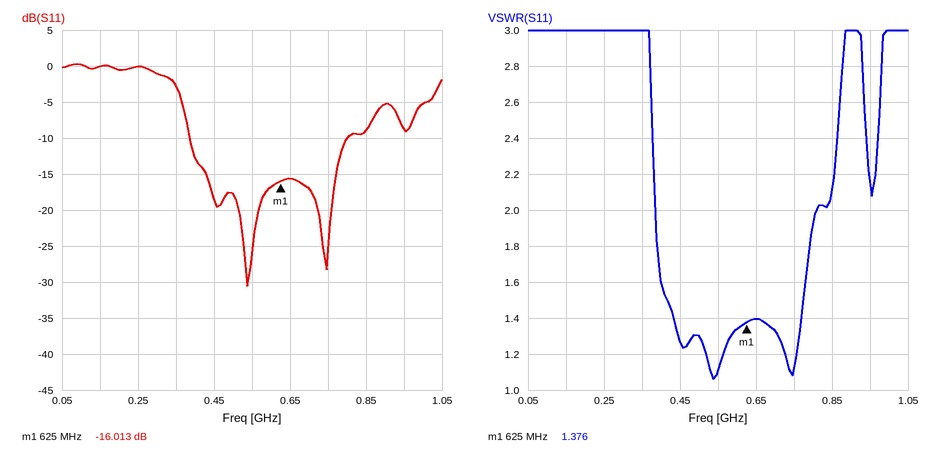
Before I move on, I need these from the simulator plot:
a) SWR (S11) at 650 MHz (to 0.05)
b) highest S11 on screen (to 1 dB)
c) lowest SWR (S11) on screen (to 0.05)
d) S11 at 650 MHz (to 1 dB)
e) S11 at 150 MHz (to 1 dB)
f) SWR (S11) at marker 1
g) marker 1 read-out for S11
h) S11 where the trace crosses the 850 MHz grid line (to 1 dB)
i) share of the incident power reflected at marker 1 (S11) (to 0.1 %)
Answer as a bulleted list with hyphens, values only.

- 1.40
- 0 dB
- 1.05
- -16 dB
- 0 dB
- 1.376
- -16.013 dB
- -9 dB
- 2.5 %
